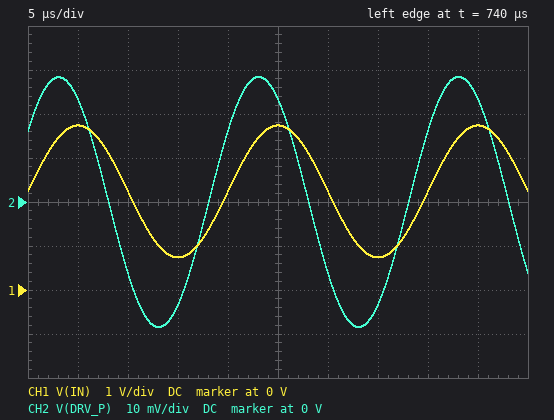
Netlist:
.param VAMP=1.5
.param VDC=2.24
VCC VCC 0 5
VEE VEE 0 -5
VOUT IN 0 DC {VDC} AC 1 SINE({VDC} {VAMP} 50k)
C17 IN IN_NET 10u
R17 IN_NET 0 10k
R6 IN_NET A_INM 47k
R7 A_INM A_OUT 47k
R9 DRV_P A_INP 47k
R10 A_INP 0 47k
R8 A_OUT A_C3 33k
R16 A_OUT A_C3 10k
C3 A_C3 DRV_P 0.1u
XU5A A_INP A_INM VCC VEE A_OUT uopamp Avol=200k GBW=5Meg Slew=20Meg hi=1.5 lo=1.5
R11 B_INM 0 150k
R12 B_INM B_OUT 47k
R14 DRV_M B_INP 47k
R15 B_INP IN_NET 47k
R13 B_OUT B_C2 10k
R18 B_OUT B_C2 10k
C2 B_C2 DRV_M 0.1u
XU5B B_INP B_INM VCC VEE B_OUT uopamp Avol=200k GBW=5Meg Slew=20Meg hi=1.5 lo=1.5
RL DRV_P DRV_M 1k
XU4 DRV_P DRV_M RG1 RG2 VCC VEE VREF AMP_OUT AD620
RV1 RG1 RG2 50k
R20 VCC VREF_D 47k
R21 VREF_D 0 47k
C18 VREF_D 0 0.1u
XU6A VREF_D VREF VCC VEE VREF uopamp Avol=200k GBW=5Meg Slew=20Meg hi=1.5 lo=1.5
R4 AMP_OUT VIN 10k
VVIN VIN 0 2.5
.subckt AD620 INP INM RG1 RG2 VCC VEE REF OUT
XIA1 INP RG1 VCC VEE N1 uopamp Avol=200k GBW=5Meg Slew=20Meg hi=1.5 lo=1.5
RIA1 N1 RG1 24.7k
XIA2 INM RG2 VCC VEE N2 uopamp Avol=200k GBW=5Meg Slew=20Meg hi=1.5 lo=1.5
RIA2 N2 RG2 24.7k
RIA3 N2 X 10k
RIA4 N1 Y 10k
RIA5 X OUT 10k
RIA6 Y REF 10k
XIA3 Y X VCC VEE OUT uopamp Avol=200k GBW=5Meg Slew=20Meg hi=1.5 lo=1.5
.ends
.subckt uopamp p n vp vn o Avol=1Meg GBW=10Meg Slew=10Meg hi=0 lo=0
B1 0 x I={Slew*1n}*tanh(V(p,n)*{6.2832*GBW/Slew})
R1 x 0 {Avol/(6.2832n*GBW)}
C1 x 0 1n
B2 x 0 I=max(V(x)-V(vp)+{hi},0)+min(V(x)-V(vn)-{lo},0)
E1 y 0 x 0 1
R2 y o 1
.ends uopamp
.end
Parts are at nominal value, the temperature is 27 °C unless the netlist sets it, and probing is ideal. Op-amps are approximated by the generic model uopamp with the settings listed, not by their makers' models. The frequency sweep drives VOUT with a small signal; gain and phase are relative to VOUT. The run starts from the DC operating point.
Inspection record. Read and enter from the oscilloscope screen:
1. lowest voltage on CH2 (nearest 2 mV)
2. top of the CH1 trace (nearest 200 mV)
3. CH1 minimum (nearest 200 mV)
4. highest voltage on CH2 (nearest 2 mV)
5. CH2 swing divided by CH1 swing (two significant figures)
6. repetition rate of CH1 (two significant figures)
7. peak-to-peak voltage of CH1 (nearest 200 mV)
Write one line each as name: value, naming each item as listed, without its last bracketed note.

lowest voltage on CH2: -28 mV
top of the CH1 trace: 3.8 V
CH1 minimum: 800 mV
highest voltage on CH2: 28 mV
CH2 swing divided by CH1 swing: 0.019
repetition rate of CH1: 50 kHz
peak-to-peak voltage of CH1: 3.0 V
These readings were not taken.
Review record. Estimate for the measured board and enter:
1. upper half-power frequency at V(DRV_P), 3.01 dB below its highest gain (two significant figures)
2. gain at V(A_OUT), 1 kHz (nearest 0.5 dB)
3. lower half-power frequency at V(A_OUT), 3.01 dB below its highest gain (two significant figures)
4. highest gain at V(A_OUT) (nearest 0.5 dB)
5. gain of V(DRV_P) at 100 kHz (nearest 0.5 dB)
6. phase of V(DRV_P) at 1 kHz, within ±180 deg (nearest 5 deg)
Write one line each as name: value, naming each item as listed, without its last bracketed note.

upper half-power frequency at V(DRV_P), 3.01 dB below its highest gain: 200 Hz
gain at V(A_OUT), 1 kHz: 0 dB
lower half-power frequency at V(A_OUT), 3.01 dB below its highest gain: 45 Hz
highest gain at V(A_OUT): 3.0 dB
gain of V(DRV_P) at 100 kHz: -32.0 dB
phase of V(DRV_P) at 1 kHz, within ±180 deg: 100 deg
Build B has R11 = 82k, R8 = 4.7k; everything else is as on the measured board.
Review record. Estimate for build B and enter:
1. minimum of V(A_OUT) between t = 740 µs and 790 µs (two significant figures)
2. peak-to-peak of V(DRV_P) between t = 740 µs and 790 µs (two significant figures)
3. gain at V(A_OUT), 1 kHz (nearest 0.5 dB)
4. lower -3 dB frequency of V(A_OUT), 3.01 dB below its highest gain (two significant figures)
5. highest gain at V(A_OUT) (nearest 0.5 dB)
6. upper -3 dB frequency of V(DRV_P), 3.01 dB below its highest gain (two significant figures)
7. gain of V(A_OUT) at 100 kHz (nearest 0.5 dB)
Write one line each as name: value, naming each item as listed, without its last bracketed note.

minimum of V(A_OUT) between t = 740 µs and 790 µs: -3.5 V
peak-to-peak of V(DRV_P) between t = 740 µs and 790 µs: 5.0 V
gain at V(A_OUT), 1 kHz: 10.0 dB
lower -3 dB frequency of V(A_OUT), 3.01 dB below its highest gain: 440 Hz
highest gain at V(A_OUT): 11.0 dB
upper -3 dB frequency of V(DRV_P), 3.01 dB below its highest gain: 320 kHz
gain of V(A_OUT) at 100 kHz: 10.5 dB
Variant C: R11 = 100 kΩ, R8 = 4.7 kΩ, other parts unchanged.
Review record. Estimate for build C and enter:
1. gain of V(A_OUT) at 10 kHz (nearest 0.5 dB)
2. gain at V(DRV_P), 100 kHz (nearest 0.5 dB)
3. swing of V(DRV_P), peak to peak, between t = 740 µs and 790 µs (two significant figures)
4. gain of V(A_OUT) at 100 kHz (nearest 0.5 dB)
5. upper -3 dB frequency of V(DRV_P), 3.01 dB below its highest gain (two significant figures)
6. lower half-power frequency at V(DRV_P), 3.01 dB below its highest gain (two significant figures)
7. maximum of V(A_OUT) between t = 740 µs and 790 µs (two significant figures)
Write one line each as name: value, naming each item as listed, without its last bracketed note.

gain of V(A_OUT) at 10 kHz: 10.5 dB
gain at V(DRV_P), 100 kHz: 7.0 dB
swing of V(DRV_P), peak to peak, between t = 740 µs and 790 µs: 4.9 V
gain of V(A_OUT) at 100 kHz: 10.0 dB
upper -3 dB frequency of V(DRV_P), 3.01 dB below its highest gain: 370 kHz
lower half-power frequency at V(DRV_P), 3.01 dB below its highest gain: 450 Hz
maximum of V(A_OUT) between t = 740 µs and 790 µs: 3.5 V
